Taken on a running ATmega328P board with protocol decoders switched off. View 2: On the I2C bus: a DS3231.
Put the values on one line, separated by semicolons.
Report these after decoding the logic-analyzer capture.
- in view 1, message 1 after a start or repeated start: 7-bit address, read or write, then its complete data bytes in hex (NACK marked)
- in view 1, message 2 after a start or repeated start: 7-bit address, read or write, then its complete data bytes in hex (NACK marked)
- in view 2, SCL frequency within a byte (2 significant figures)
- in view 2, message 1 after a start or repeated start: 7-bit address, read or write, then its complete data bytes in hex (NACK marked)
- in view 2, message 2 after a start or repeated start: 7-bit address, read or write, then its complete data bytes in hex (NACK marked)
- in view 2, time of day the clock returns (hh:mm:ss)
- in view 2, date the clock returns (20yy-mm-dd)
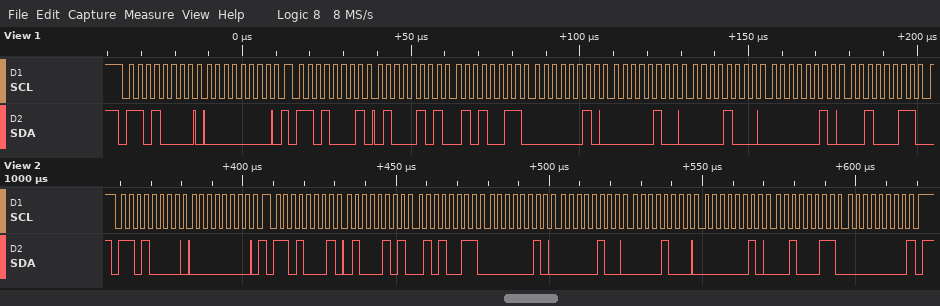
0x68 write: 00; 0x68 read: 45 53 02 04 08 02 23; 400 kHz; 0x68 write: 00; 0x68 read: 45 53 02 04 08 02 23 00 NACK; 02:53:45; 2023-02-08
